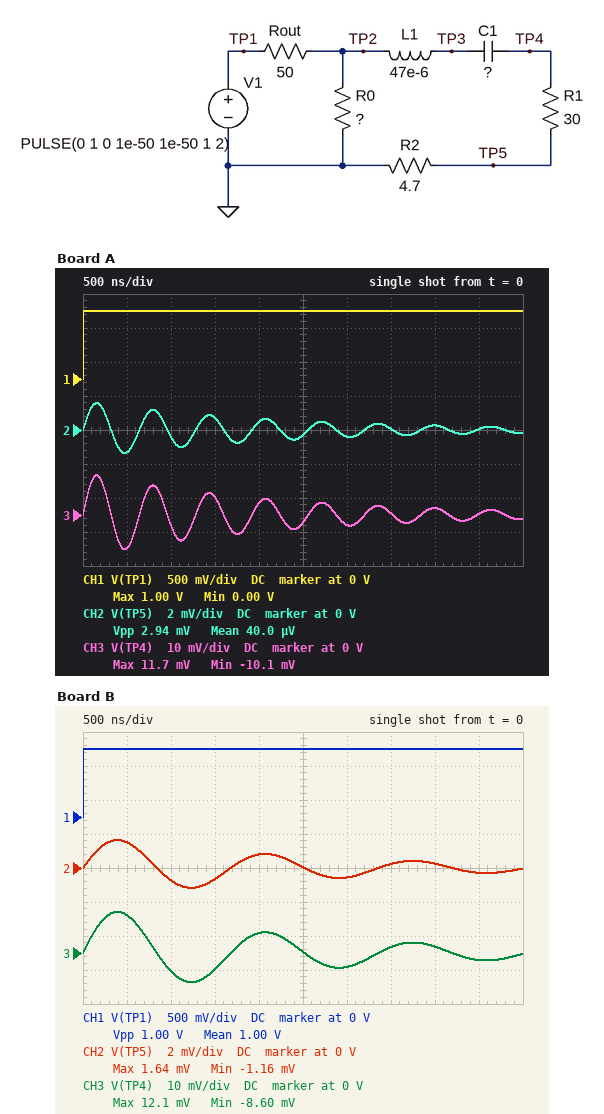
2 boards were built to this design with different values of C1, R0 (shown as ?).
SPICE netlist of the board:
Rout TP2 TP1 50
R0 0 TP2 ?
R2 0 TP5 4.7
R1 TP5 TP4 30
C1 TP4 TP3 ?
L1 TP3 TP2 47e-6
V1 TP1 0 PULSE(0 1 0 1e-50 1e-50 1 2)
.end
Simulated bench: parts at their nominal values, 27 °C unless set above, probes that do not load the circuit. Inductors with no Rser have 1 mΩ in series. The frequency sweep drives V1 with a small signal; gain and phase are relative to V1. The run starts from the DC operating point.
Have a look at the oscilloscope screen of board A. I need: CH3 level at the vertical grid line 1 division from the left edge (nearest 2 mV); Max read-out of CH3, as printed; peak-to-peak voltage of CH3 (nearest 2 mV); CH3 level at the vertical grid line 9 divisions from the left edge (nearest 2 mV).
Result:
-10 mV
11.7 mV
22 mV
0 V
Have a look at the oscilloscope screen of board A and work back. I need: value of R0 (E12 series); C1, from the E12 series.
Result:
10 Ω
220 pF
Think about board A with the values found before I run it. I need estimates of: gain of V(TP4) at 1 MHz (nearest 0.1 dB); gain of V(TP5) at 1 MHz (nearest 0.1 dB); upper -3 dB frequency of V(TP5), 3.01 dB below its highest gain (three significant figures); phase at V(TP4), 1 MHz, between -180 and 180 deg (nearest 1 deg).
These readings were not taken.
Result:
-37.4 dB
-54.8 dB
1.64 MHz
84 deg
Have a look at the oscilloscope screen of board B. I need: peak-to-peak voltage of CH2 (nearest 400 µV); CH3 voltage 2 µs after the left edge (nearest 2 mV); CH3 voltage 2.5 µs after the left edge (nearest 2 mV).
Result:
2.8 mV
6 mV
0 V
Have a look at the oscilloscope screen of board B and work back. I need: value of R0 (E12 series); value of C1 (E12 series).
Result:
3.9 Ω
1.5 nF
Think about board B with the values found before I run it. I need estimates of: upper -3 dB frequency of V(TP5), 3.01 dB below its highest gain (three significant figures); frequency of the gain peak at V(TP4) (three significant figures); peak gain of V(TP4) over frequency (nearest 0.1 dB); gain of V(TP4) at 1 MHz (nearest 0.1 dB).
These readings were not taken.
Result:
668 kHz
599 kHz
-23.7 dB
-37.7 dB
